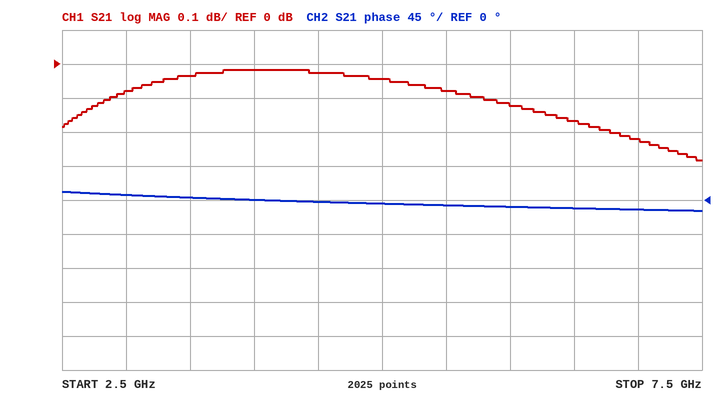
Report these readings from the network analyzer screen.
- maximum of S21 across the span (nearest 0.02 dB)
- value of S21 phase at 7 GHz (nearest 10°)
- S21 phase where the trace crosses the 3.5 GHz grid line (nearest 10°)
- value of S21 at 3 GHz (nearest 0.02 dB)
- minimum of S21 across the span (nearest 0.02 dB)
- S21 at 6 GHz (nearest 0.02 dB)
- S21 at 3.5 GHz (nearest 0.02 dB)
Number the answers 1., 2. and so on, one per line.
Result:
1. -0.02 dB
2. -10°
3. 0°
4. -0.08 dB
5. -0.28 dB
6. -0.12 dB
7. -0.04 dB
